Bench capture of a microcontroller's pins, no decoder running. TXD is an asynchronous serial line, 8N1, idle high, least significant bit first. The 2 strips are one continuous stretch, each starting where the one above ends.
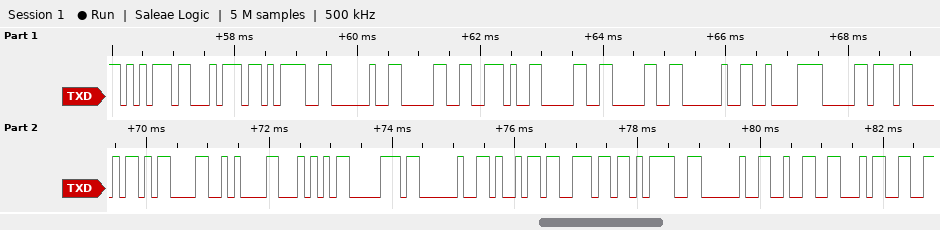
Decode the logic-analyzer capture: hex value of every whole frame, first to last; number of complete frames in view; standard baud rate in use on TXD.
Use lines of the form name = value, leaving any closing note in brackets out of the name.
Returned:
hex value of every whole frame, first to last = 75 74 3D 20 30 2E 30 30 20 C2 B0 43 0D 0A 54 70 20 69 6E 3D 20 32 34
number of complete frames in view = 23
standard baud rate in use on TXD = 9600 baud
